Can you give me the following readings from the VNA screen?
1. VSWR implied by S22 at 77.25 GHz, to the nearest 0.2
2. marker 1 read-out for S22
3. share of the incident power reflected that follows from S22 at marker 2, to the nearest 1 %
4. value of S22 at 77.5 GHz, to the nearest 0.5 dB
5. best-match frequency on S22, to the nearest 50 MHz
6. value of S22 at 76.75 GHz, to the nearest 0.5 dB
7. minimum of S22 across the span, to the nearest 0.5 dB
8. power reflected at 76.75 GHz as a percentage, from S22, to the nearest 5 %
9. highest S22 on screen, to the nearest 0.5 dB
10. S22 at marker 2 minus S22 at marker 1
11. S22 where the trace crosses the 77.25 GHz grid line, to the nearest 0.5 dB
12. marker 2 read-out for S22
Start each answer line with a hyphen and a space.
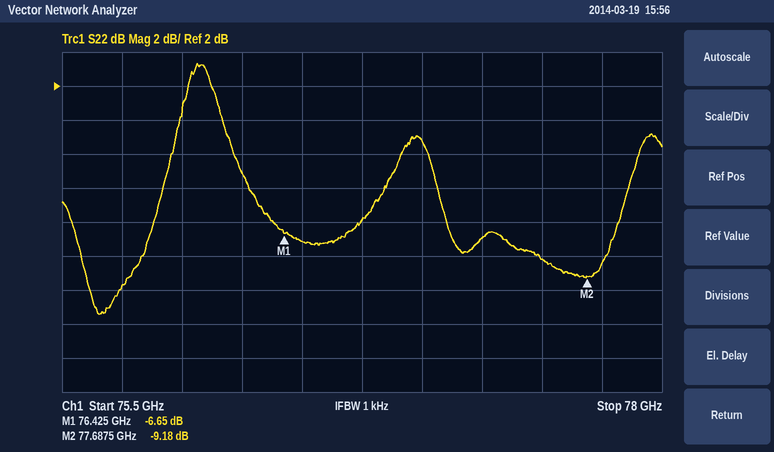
- 2.6
- -6.65 dB
- 12 %
- -8.0 dB
- 75.65 GHz
- -6.0 dB
- -11.5 dB
- 25 %
- 3.5 dB
- -2.53 dB
- -7.0 dB
- -9.18 dB
